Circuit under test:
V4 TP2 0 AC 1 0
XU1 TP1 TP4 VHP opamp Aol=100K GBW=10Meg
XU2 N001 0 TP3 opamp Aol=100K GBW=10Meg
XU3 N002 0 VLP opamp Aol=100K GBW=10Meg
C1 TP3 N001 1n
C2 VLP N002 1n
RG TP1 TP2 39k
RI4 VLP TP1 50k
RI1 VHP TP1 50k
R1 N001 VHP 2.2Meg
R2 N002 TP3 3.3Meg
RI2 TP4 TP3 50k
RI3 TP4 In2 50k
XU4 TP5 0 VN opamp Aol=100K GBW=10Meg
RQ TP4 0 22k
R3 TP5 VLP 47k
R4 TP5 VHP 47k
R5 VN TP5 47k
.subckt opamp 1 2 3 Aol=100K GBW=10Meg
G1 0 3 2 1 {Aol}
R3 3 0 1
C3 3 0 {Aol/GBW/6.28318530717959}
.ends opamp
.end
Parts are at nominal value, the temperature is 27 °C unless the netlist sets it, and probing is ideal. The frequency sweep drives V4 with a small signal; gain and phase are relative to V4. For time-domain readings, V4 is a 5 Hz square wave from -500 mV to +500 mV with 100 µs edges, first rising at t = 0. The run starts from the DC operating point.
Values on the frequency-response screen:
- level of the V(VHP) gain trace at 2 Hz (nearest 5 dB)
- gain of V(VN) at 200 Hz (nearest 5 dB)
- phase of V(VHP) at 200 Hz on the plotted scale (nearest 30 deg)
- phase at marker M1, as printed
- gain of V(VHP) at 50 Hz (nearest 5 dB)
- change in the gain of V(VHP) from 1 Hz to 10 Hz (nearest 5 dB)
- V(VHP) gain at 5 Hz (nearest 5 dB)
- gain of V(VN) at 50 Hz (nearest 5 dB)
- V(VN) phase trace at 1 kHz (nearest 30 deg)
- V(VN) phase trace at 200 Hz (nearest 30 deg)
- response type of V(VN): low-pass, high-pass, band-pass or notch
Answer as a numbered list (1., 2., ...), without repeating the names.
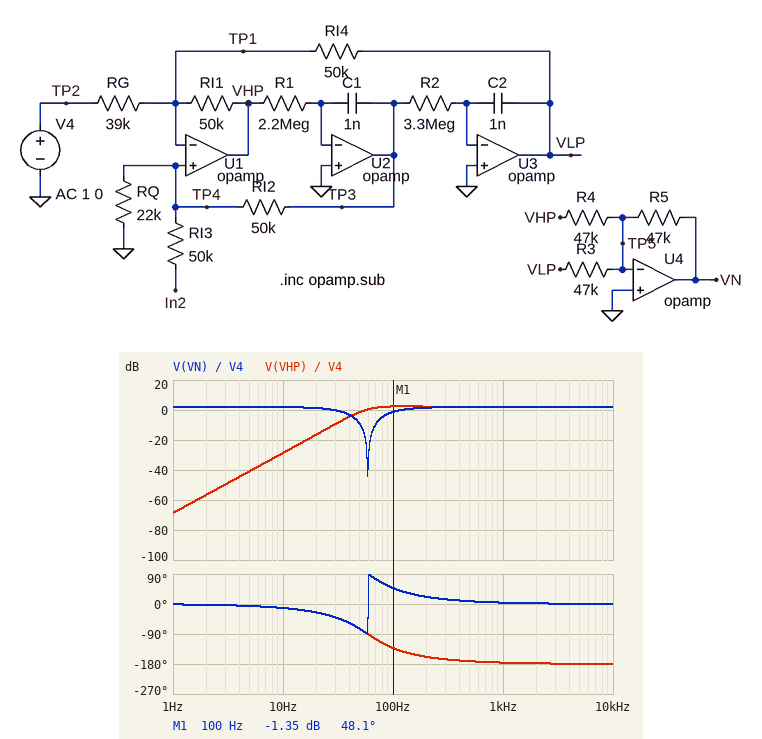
1. -55 dB
2. 0 dB
3. -150 deg
4. 48.1 deg
5. 0 dB
6. 40 dB
7. -40 dB
8. -10 dB
9. 0 deg
10. 30 deg
11. notch
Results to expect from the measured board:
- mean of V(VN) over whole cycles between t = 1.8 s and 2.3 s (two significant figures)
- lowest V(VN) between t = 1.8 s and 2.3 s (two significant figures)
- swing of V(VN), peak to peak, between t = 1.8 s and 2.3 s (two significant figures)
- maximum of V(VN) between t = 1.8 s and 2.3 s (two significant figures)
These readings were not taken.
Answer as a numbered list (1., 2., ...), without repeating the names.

1. 120 mV
2. -710 mV
3. 1.4 V
4. 710 mV
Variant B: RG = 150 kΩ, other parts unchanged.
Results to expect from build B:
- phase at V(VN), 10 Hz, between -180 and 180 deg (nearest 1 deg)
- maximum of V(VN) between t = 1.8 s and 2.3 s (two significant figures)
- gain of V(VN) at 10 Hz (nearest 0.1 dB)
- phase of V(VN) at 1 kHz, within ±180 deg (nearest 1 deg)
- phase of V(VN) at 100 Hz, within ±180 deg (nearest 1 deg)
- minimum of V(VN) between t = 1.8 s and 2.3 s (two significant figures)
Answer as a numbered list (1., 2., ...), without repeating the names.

1. -9 deg
2. 200 mV
3. -9.6 dB
4. 3 deg
5. 38 deg
6. -200 mV
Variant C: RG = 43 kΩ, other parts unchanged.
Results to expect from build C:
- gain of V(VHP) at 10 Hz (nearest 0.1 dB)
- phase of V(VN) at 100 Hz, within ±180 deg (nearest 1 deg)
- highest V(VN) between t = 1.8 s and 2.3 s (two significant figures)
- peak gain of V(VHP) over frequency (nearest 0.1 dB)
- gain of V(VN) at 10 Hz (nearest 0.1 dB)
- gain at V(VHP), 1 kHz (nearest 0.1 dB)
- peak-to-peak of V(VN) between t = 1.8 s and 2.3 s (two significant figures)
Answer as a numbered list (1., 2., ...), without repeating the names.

1. -29.5 dB
2. 47 deg
3. 650 mV
4. 1.7 dB
5. 1.1 dB
6. 1.3 dB
7. 1.3 V
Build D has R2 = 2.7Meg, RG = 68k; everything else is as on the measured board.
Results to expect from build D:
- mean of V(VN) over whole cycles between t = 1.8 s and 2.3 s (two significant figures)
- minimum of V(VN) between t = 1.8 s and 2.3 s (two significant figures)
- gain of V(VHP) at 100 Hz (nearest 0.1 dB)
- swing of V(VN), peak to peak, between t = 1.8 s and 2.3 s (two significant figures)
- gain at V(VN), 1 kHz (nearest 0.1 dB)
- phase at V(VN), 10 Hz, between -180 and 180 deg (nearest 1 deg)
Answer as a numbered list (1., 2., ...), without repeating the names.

1. 68 mV
2. -440 mV
3. -1.1 dB
4. 890 mV
5. -2.7 dB
6. -8 deg
